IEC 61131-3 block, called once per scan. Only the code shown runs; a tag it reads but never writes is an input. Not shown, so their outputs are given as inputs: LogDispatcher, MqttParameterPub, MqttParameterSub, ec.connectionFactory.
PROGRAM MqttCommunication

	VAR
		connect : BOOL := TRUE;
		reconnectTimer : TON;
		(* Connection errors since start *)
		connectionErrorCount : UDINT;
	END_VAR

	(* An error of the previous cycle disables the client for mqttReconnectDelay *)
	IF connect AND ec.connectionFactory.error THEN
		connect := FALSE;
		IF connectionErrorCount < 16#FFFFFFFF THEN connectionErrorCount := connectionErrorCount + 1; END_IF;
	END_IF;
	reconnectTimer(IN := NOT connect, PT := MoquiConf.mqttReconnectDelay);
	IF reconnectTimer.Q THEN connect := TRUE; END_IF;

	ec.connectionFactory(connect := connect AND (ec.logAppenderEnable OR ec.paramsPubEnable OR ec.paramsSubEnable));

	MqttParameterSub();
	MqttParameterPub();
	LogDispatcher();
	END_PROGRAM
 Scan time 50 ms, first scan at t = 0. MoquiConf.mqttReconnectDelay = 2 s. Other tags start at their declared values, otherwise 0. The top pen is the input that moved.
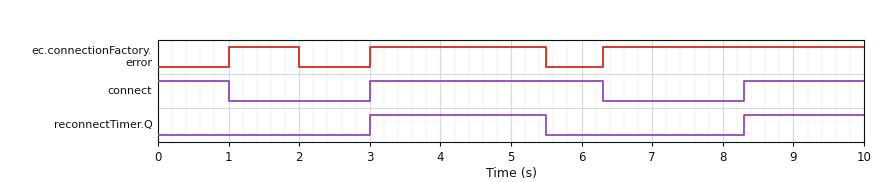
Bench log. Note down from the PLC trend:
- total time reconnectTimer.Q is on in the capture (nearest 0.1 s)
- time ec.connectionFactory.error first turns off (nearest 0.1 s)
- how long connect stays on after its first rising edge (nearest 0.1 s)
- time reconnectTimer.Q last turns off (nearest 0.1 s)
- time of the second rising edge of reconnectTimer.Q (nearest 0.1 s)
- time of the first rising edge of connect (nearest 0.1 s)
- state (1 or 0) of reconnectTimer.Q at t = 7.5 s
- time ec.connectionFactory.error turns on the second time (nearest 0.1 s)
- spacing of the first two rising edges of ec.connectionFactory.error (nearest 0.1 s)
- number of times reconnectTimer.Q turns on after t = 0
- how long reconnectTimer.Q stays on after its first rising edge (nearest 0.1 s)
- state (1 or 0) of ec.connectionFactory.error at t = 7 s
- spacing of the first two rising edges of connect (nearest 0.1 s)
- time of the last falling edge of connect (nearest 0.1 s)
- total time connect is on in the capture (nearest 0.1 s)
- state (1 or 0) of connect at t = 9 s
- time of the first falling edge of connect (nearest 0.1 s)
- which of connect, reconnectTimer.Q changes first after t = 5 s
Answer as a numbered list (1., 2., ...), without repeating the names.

1. 4.2 s
2. 2.0 s
3. 3.3 s
4. 5.5 s
5. 8.3 s
6. 3.0 s
7. 0
8. 3.0 s
9. 2.0 s
10. 2
11. 2.5 s
12. 1
13. 5.3 s
14. 6.3 s
15. 6.0 s
16. 1
17. 1.0 s
18. reconnectTimer.Q
